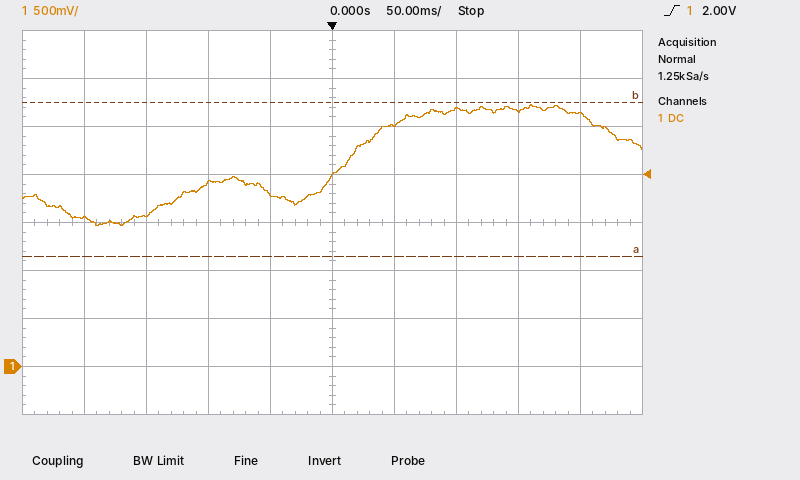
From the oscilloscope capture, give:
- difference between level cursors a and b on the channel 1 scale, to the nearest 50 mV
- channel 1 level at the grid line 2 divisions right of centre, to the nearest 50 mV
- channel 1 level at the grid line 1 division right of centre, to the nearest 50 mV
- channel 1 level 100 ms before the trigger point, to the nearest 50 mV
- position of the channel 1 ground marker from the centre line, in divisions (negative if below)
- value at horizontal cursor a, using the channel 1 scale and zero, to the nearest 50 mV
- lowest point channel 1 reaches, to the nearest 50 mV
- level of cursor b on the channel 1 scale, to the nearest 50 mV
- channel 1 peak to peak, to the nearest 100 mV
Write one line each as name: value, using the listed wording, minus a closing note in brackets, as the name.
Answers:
difference between level cursors a and b on the channel 1 scale, to the nearest 50 mV: 1.60 V
channel 1 level at the grid line 2 divisions right of centre, to the nearest 50 mV: 2.70 V
channel 1 level at the grid line 1 division right of centre, to the nearest 50 mV: 2.50 V
channel 1 level 100 ms before the trigger point, to the nearest 50 mV: 1.90 V
position of the channel 1 ground marker from the centre line, in divisions: -3.0 div
value at horizontal cursor a, using the channel 1 scale and zero, to the nearest 50 mV: 1.15 V
lowest point channel 1 reaches, to the nearest 50 mV: 1.45 V
level of cursor b on the channel 1 scale, to the nearest 50 mV: 2.75 V
channel 1 peak to peak, to the nearest 100 mV: 1.30 V
